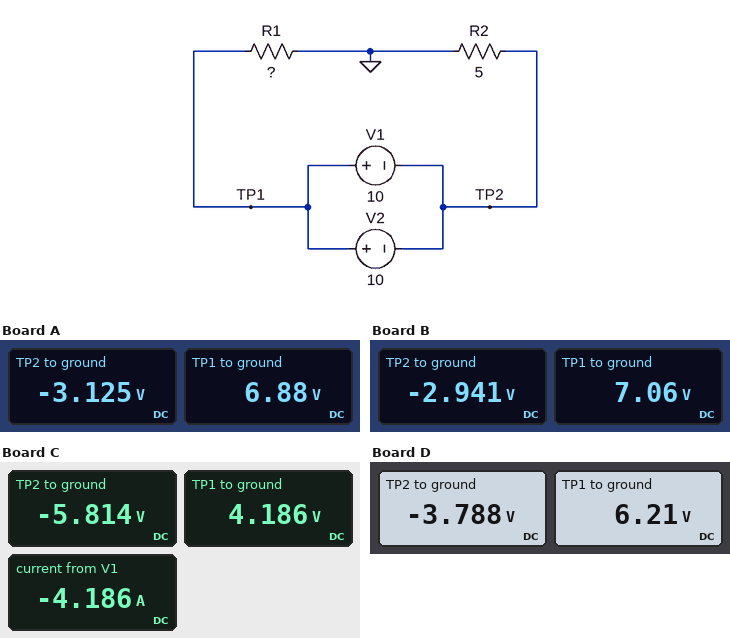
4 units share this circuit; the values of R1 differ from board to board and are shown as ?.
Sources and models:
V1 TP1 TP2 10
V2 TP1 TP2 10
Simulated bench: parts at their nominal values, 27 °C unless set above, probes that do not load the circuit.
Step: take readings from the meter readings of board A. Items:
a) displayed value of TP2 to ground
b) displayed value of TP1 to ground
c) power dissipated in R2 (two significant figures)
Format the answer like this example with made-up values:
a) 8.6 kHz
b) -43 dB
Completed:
a) -3.125 V
b) 6.88 V
c) 2.0 W
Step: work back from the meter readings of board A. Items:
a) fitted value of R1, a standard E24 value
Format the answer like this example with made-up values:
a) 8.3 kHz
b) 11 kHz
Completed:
a) 11 Ω
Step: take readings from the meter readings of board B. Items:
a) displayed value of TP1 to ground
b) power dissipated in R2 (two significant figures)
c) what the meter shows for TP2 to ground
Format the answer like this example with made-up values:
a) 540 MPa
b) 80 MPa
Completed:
a) 7.06 V
b) 1.7 W
c) -2.941 V
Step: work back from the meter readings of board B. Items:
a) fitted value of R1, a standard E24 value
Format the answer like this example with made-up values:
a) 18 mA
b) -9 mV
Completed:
a) 12 Ω
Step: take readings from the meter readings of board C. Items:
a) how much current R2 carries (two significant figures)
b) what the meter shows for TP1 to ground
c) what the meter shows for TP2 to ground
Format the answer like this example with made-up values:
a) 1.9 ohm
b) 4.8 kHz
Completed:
a) 1.2 A
b) 4.186 V
c) -5.814 V
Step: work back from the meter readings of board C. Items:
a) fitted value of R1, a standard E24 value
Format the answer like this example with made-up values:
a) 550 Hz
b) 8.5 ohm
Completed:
a) 3.6 Ω
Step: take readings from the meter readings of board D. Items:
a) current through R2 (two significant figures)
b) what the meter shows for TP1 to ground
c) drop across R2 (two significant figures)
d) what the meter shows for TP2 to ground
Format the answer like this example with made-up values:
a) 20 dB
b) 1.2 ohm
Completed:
a) 760 mA
b) 6.21 V
c) 3.8 V
d) -3.788 V
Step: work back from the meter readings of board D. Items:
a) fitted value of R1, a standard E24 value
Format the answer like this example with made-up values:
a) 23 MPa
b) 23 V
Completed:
a) 8.2 Ω
